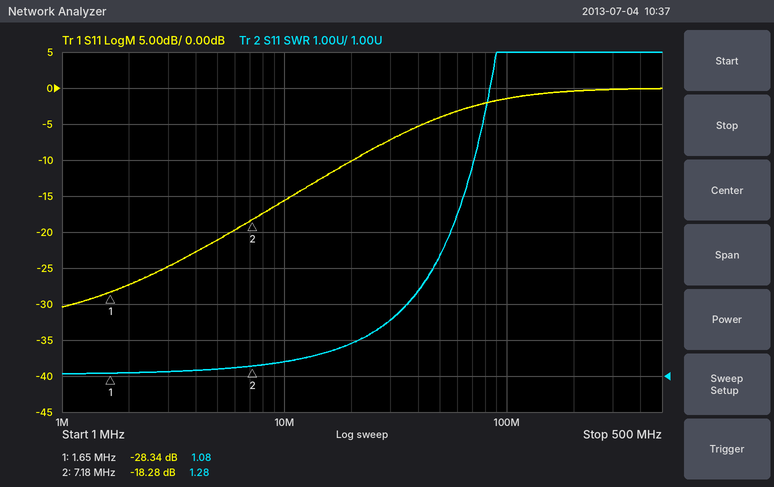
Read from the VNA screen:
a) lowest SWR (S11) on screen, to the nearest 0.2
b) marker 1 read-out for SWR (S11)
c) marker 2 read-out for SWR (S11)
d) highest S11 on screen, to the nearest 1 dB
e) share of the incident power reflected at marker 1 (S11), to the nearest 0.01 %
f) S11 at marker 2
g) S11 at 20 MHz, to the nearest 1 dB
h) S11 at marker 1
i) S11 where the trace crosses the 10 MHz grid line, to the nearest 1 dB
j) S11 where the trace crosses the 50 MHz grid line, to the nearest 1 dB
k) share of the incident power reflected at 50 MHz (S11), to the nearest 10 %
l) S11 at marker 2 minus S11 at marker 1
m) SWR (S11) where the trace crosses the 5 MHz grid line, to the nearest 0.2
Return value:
1.0
1.08
1.28
0 dB
0.15 %
-18.28 dB
-10 dB
-28.34 dB
-16 dB
-4 dB
40 %
10.06 dB
1.2
